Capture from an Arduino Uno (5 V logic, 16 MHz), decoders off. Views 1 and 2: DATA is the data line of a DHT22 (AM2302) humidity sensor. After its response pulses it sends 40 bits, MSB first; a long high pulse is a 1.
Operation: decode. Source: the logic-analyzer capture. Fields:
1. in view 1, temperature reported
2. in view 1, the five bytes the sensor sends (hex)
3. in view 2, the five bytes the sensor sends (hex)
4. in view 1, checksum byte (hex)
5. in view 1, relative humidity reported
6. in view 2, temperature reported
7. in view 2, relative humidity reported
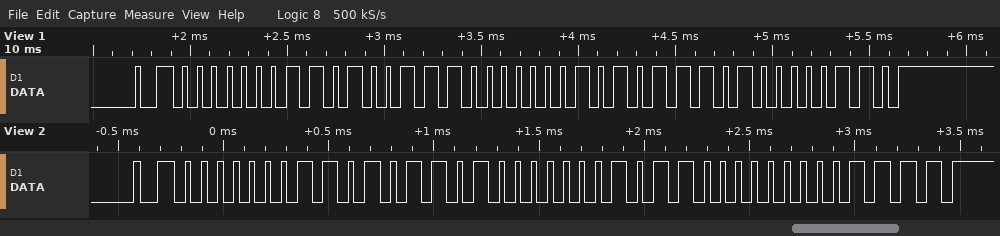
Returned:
34.9 °C
01 A7 01 5D 06
01 AD 01 60 0F
0x06
42.3 %
35.2 °C
42.9 %
